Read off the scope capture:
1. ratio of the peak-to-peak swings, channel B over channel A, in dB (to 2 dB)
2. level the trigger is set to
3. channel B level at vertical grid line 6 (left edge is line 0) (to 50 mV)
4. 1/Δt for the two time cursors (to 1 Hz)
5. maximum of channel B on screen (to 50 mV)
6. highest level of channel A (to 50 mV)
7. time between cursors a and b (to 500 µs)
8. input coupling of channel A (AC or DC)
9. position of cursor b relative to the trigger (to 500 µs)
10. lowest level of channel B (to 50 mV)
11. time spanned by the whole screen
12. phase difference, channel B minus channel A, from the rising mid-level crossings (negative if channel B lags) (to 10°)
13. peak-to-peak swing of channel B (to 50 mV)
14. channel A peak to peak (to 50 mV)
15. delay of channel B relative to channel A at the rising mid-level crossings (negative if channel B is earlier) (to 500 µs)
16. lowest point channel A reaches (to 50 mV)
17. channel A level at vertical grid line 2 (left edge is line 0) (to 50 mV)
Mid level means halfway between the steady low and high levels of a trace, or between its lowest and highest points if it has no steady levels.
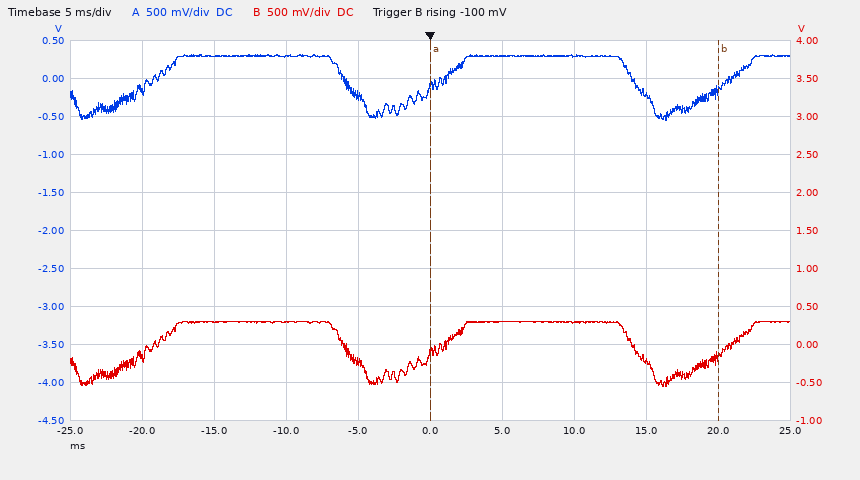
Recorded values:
0 dB
-100 mV
300 mV
50 Hz
300 mV
300 mV
20.0 ms
DC
+20.0 ms
-550 mV
50 ms
0°
850 mV
850 mV
0.0 ms
-550 mV
300 mV
